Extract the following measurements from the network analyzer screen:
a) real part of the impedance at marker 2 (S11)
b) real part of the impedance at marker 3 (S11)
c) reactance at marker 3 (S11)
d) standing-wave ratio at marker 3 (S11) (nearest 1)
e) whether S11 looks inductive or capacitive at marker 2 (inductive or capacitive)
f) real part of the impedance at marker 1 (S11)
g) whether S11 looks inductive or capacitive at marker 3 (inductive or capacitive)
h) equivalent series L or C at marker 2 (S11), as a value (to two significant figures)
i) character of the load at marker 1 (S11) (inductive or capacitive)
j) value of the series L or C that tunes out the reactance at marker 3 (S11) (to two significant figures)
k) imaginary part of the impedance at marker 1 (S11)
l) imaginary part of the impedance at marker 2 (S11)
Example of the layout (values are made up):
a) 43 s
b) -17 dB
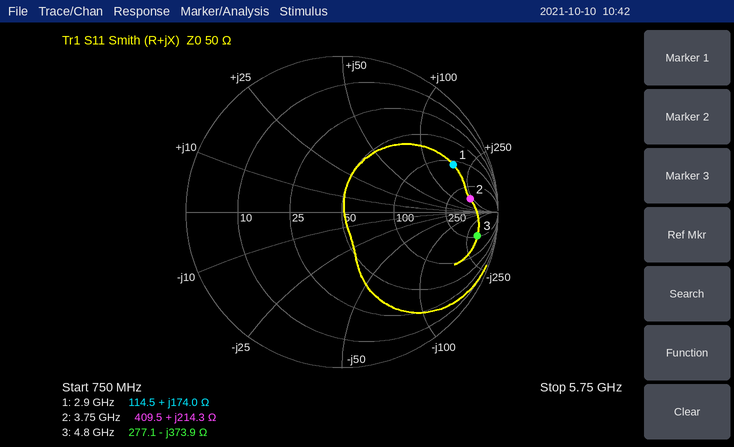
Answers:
a) 409.5 Ω
b) 277.1 Ω
c) -373.9 Ω
d) 16
e) inductive
f) 114.5 Ω
g) capacitive
h) 9.1 nH
i) inductive
j) 12 nH
k) +174.0 Ω
l) +214.3 Ω
